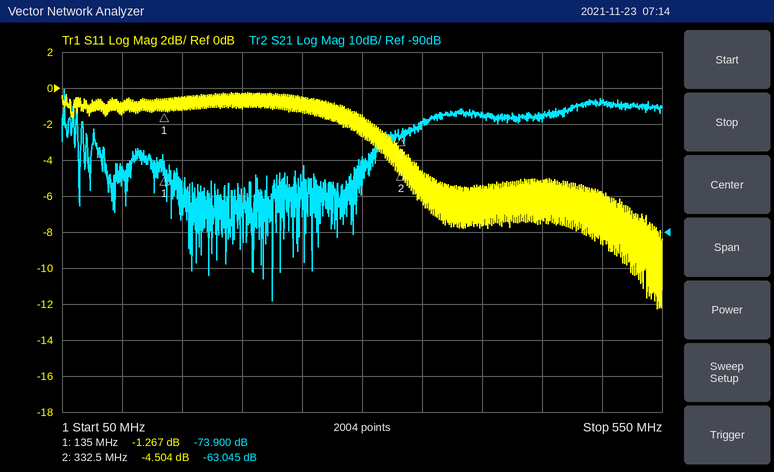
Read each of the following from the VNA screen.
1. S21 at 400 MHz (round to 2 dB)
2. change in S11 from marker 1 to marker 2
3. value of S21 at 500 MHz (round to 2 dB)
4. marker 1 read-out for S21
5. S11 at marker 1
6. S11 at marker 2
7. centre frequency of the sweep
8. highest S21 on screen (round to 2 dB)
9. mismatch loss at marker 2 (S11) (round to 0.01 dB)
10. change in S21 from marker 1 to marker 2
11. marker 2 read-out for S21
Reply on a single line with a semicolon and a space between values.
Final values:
-58 dB; -3.237 dB; -54 dB; -73.900 dB; -1.267 dB; -4.504 dB; 300 MHz; -50 dB; 1.90 dB; 10.855 dB; -63.045 dB
